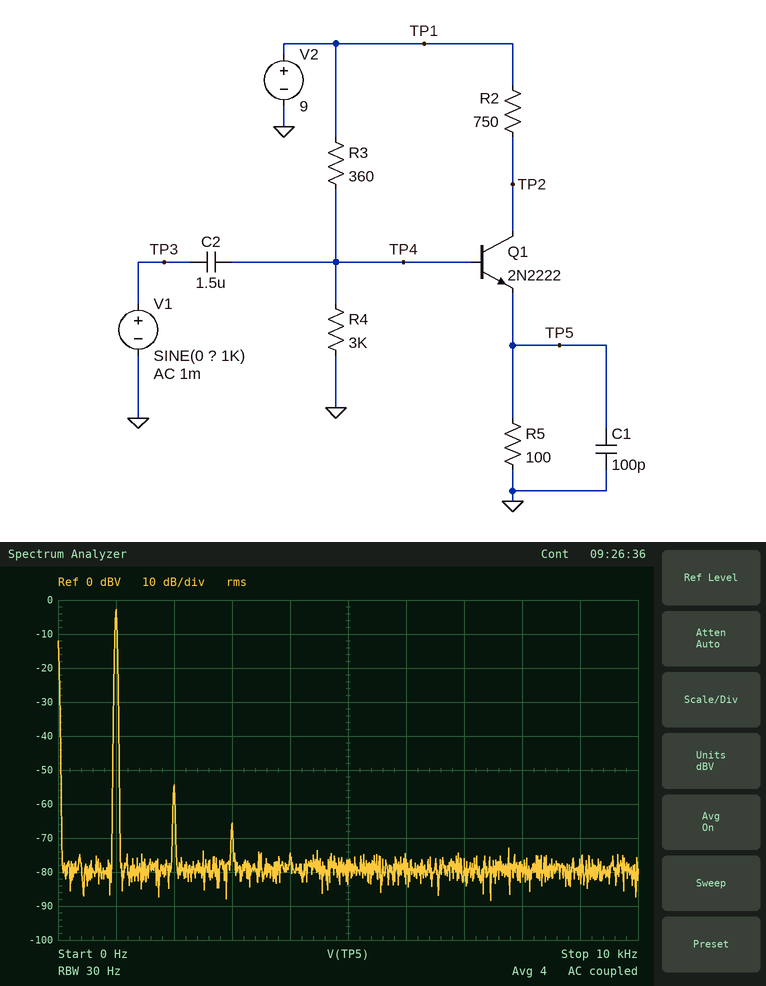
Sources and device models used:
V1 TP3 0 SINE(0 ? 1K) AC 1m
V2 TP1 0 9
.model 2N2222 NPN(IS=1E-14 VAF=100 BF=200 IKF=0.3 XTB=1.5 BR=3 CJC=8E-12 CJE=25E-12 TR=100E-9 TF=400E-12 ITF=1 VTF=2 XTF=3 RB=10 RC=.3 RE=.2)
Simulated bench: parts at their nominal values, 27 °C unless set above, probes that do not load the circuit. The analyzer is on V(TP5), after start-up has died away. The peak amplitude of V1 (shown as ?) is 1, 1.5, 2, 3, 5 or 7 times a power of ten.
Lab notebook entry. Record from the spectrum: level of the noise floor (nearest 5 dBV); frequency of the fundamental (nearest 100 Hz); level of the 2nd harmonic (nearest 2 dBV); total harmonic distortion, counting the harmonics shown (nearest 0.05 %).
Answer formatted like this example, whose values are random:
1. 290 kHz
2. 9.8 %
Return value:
1. -80 dBV
2. 1.0 kHz
3. -54 dBV
4. 0.25 %
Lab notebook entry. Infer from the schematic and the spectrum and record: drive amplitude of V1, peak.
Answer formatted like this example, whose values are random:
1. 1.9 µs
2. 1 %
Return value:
1. 2 V
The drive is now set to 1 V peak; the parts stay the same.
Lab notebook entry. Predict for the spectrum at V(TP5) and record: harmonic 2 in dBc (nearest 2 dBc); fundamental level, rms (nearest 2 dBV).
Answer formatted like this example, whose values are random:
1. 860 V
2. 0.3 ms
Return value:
1. -60 dBc
2. -8 dBV
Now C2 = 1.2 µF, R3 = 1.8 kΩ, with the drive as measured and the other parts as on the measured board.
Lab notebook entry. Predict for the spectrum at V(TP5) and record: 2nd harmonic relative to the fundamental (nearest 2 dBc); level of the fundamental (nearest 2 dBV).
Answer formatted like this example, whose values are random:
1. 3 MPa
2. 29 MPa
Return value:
1. -16 dBc
2. -2 dBV
